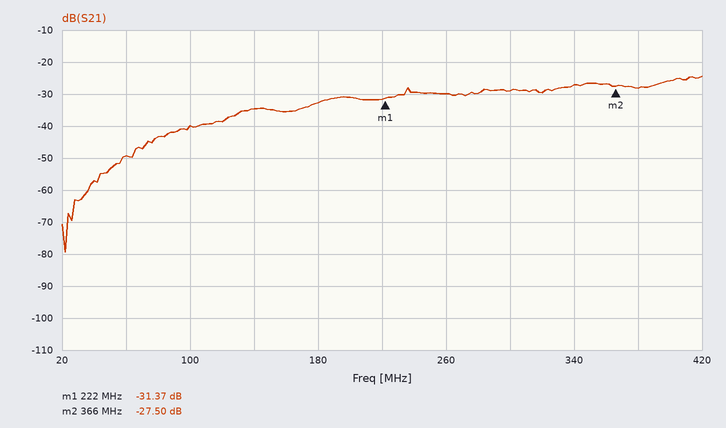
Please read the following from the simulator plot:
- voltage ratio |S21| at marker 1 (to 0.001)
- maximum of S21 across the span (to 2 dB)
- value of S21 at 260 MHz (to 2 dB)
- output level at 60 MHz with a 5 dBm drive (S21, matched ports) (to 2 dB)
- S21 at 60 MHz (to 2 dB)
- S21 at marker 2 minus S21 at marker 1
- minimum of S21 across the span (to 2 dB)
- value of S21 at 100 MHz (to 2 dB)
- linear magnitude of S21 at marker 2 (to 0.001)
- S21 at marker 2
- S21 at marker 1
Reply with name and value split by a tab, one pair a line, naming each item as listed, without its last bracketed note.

voltage ratio |S21| at marker 1	0.027
maximum of S21 across the span	-24 dB
value of S21 at 260 MHz	-30 dB
output level at 60 MHz with a 5 dBm drive (S21, matched ports)	-44 dBm
S21 at 60 MHz	-50 dB
S21 at marker 2 minus S21 at marker 1	3.87 dB
minimum of S21 across the span	-80 dB
value of S21 at 100 MHz	-40 dB
linear magnitude of S21 at marker 2	0.042
S21 at marker 2	-27.50 dB
S21 at marker 1	-31.37 dB
